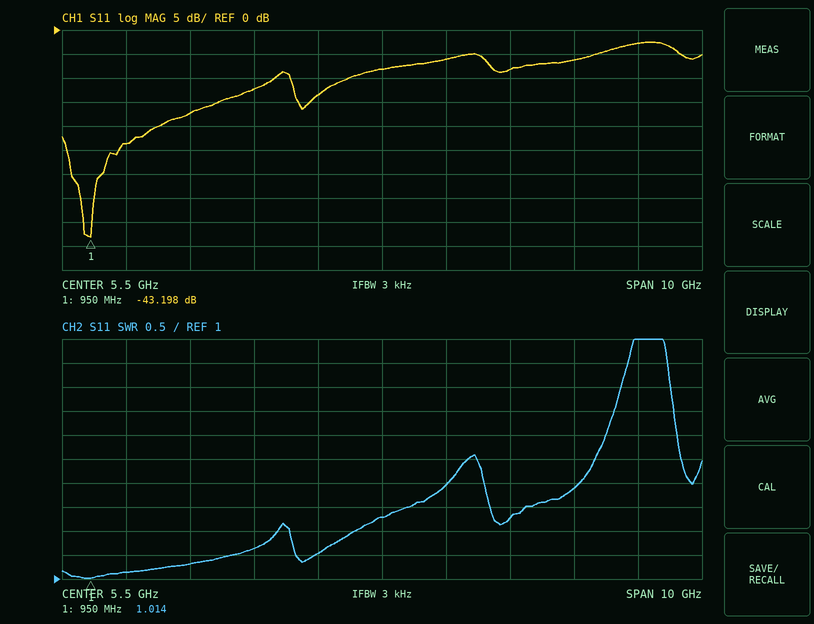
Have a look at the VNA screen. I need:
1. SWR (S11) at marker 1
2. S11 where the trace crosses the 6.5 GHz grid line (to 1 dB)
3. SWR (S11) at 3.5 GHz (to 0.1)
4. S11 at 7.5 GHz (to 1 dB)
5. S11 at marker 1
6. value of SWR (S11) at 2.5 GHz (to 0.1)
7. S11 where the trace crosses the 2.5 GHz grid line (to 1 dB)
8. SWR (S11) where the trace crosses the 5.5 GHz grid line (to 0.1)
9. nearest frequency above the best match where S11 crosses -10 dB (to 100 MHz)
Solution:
1.014
-6 dB
1.6
-8 dB
-43.198 dB
1.3
-17 dB
2.3
3.8 GHz
